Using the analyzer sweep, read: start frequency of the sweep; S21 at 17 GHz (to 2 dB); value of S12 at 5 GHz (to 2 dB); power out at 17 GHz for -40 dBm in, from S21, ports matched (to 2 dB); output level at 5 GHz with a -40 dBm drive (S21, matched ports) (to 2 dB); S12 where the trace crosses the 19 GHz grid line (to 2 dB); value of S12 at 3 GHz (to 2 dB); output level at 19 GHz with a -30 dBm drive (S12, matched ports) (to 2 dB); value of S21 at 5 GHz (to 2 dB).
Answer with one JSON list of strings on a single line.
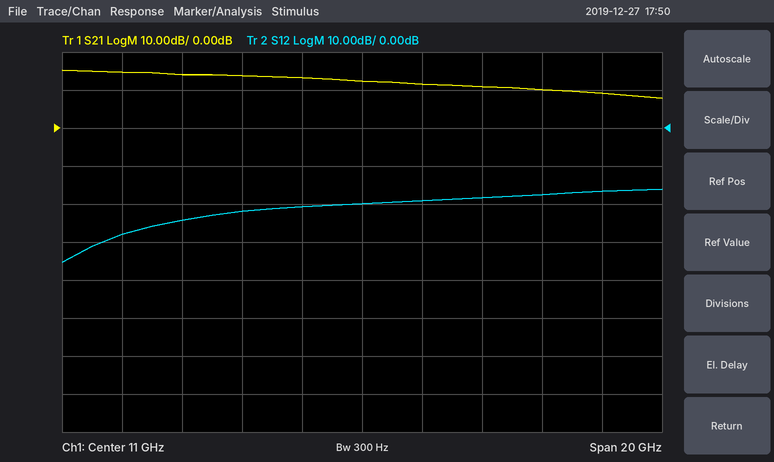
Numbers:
["1 GHz", "10 dB", "-24 dB", "-30 dBm", "-26 dBm", "-16 dB", "-28 dB", "-46 dBm", "14 dB"]
